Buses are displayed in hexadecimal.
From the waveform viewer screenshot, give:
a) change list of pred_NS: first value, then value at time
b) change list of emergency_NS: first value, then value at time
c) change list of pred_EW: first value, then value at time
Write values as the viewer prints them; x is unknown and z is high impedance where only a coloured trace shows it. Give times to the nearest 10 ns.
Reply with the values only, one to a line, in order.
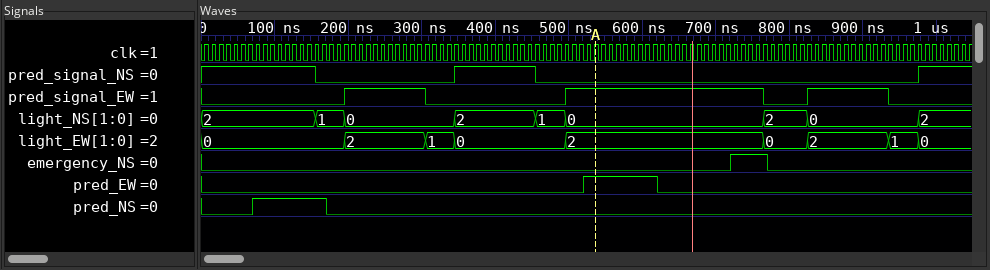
0, 1 at 70 ns, 0 at 170 ns
0, 1 at 720 ns, 0 at 770 ns
0, 1 at 520 ns, 0 at 620 ns
